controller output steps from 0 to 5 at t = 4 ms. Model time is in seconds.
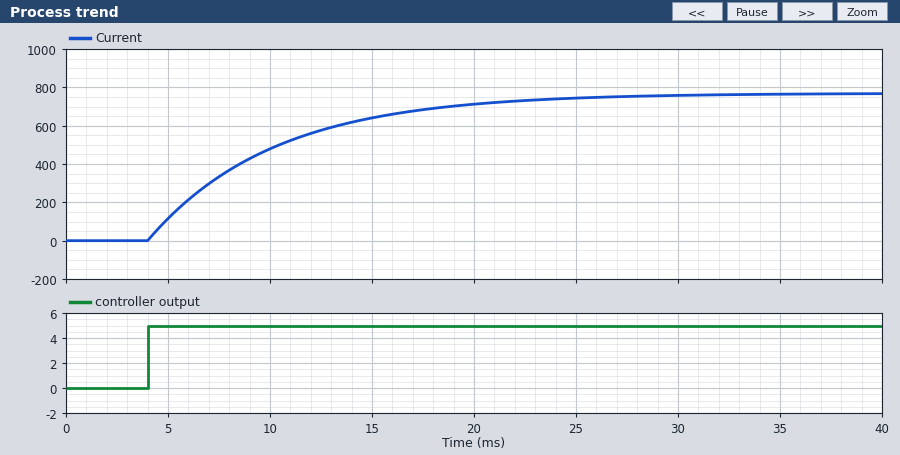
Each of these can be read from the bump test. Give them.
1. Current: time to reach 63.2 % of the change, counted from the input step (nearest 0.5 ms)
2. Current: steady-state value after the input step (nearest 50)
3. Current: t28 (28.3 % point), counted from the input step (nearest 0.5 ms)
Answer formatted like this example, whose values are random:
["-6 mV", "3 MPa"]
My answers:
["6.0 ms", "750", "2.0 ms"]
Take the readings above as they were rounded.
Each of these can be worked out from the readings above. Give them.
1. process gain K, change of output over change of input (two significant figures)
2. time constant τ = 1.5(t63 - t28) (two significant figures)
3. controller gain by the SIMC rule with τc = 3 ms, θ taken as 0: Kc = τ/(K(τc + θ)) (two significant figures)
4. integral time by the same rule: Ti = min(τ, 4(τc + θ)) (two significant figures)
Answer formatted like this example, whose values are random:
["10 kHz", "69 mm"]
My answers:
["150", "6.0 ms", "0.013", "6.0 ms"]
